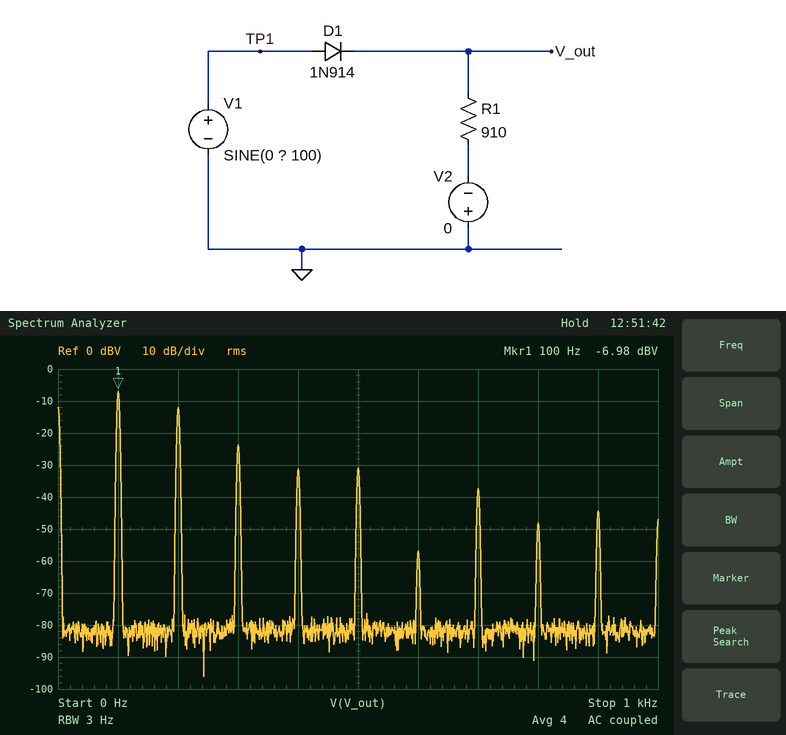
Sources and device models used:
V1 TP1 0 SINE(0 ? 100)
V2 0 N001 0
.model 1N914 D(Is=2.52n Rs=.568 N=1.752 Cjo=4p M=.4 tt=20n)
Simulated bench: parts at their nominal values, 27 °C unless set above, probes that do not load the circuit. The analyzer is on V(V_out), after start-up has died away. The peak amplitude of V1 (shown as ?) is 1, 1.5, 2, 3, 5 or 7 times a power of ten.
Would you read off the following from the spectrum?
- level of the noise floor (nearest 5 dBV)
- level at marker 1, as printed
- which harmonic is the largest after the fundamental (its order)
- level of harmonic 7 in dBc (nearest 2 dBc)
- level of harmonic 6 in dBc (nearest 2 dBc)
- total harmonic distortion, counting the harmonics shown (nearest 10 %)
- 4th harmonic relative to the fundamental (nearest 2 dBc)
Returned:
-80 dBV
-6.98 dBV
2
-30 dBc
-50 dBc
60 %
-24 dBc
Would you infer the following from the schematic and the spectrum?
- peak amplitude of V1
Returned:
2 V
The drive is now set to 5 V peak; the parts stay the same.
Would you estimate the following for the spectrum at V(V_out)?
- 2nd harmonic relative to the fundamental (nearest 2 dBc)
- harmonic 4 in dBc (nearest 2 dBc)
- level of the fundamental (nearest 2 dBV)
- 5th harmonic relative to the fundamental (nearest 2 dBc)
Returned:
-6 dBc
-22 dBc
4 dBV
-30 dBc
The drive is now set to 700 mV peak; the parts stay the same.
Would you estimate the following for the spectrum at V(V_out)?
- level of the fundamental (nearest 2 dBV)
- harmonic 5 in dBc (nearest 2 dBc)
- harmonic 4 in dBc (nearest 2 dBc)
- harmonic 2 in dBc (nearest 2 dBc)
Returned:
-26 dBV
-34 dBc
-14 dBc
-2 dBc
